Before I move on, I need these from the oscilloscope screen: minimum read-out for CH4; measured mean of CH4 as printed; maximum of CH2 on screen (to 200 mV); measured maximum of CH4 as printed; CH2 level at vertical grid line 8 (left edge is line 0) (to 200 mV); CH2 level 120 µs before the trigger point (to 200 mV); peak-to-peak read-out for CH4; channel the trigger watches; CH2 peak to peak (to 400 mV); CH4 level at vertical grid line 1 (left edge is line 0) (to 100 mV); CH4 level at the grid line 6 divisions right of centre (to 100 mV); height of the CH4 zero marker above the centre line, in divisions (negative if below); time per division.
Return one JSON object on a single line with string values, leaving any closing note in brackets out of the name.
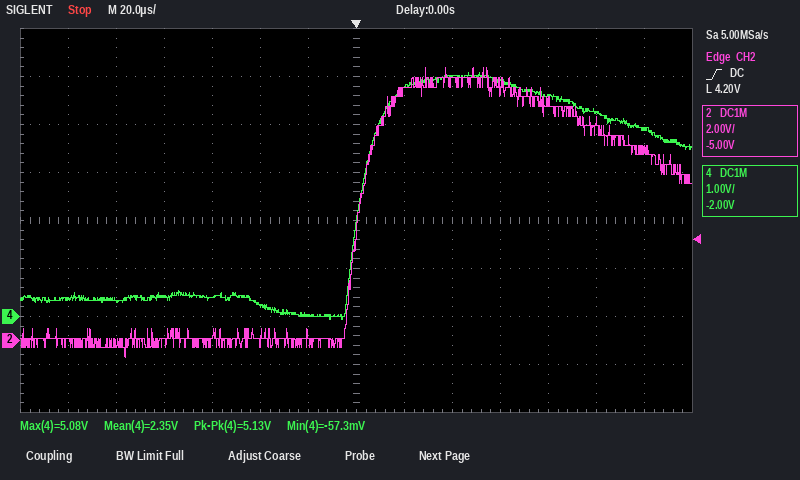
{"minimum read-out for CH4": "-57.3 mV", "measured mean of CH4 as printed": "2.35 V", "maximum of CH2 on screen": "11.4 V", "measured maximum of CH4 as printed": "5.08 V", "CH2 level at vertical grid line 8 (left edge is line 0)": "10.4 V", "CH2 level 120 µs before the trigger point": "0.0 V", "peak-to-peak read-out for CH4": "5.13 V", "channel the trigger watches": "CH2", "CH2 peak to peak": "12.0 V", "CH4 level at vertical grid line 1 (left edge is line 0)": "400 mV", "CH4 level at the grid line 6 divisions right of centre": "3.9 V", "height of the CH4 zero marker above the centre line, in divisions": "-2.0 div", "time per division": "20 µs"}
